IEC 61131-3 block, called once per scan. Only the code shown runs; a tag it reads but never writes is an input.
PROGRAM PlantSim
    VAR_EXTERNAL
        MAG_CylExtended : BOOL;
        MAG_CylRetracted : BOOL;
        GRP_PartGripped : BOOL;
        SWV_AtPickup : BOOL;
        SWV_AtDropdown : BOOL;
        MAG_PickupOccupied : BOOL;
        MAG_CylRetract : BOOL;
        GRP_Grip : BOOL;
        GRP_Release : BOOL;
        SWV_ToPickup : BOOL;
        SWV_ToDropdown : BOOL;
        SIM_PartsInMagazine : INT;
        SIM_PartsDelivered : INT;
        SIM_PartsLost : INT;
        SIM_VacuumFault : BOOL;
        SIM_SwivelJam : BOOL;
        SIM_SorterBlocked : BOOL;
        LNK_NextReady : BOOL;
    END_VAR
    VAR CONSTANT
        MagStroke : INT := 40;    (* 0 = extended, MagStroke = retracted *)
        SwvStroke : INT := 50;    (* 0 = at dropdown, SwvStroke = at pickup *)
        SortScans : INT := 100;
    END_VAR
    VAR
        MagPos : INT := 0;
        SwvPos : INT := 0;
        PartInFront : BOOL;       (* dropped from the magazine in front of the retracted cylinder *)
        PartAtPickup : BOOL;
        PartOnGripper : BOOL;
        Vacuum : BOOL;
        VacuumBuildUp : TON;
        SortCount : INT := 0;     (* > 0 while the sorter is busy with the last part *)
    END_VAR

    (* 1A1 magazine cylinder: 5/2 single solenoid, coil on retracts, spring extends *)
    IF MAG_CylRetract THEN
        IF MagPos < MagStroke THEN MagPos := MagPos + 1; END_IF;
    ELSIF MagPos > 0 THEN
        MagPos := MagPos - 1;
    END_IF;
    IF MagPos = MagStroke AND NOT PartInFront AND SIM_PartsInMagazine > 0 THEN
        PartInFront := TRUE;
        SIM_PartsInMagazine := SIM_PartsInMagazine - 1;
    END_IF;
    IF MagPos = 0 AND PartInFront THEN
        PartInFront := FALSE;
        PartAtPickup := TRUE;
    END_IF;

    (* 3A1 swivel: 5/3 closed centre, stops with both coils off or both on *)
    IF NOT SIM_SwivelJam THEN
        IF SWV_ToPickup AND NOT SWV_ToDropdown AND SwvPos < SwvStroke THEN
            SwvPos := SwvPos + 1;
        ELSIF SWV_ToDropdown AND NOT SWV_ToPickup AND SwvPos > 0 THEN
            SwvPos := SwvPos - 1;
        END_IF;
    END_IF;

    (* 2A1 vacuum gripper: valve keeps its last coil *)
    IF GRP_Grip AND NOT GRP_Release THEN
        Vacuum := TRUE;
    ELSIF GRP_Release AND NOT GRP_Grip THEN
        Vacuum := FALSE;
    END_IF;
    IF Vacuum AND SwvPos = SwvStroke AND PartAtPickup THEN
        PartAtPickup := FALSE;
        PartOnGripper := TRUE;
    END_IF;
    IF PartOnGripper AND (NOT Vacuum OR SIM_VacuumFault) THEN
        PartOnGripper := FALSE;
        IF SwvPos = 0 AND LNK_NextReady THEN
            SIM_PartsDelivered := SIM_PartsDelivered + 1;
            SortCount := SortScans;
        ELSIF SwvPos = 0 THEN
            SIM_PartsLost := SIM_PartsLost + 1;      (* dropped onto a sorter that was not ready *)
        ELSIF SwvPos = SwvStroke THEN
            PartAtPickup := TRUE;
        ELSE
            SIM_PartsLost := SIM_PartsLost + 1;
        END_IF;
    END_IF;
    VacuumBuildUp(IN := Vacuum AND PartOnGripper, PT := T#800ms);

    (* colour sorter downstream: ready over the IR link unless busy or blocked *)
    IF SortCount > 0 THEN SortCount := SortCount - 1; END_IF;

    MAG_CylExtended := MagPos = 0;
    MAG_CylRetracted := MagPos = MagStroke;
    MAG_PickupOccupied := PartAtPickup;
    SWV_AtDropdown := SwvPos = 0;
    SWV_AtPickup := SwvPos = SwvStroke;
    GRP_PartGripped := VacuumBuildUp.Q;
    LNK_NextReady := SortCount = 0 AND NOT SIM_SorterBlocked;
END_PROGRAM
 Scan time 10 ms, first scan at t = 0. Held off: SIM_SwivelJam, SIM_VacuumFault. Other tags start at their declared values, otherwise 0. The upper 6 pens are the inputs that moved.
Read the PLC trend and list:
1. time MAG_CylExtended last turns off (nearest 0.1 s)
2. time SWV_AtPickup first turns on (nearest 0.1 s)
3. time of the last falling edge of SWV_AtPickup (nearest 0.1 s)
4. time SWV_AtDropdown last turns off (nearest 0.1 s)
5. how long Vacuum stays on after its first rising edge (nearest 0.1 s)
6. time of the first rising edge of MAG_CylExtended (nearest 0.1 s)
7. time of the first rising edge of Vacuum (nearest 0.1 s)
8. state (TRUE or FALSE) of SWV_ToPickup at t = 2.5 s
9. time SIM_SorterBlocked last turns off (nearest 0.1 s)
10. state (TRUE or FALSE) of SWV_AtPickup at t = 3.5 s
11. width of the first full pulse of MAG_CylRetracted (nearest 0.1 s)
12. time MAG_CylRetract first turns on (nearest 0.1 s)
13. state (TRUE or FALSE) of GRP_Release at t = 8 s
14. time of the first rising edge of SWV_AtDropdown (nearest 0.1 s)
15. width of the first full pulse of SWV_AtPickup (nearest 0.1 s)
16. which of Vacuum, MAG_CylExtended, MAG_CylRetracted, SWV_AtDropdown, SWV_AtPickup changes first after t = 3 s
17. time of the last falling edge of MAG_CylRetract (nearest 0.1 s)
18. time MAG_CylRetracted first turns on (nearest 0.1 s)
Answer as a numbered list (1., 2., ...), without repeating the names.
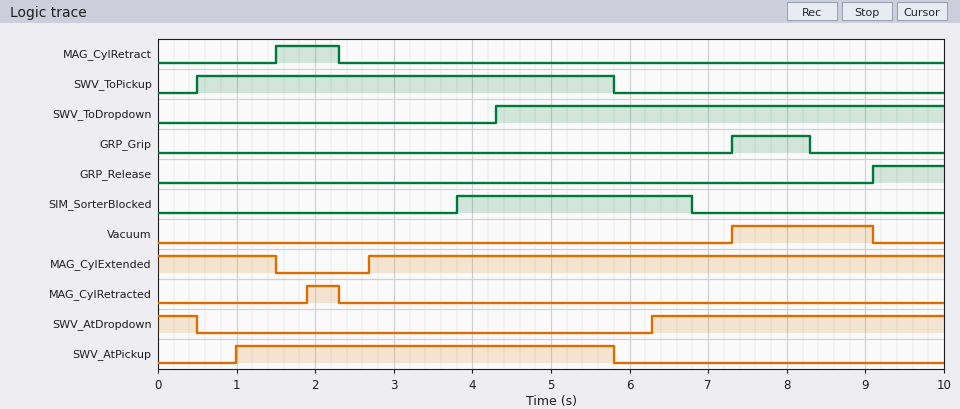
1. 1.5 s
2. 1.0 s
3. 5.8 s
4. 0.5 s
5. 1.8 s
6. 2.7 s
7. 7.3 s
8. TRUE
9. 6.8 s
10. TRUE
11. 0.4 s
12. 1.5 s
13. FALSE
14. 6.3 s
15. 4.8 s
16. SWV_AtPickup
17. 2.3 s
18. 1.9 s
